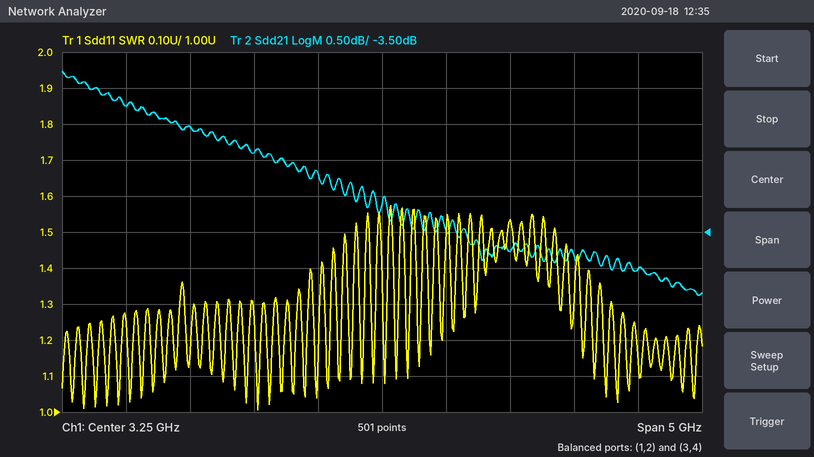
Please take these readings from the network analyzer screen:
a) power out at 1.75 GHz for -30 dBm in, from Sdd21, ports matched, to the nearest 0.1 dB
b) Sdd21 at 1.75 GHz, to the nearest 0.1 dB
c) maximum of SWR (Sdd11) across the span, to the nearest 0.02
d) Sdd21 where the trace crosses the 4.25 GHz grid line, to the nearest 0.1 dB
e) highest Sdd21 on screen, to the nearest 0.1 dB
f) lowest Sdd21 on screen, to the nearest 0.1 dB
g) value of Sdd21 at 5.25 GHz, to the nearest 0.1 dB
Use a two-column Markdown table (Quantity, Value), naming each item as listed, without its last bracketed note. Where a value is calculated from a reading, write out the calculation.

| Quantity | Value |
|---|---|
| power out at 1.75 GHz for -30 dBm in, from Sdd21, ports matched, to the nearest 0.1 dB | -30 dBm + (-2.0 dB) = -32.0 dBm |
| Sdd21 at 1.75 GHz, to the nearest 0.1 dB | -2.0 dB |
| maximum of SWR (Sdd11) across the span, to the nearest 0.02 | 1.58 |
| Sdd21 where the trace crosses the 4.25 GHz grid line, to the nearest 0.1 dB | -3.8 dB |
| highest Sdd21 on screen, to the nearest 0.1 dB | -1.3 dB |
| lowest Sdd21 on screen, to the nearest 0.1 dB | -4.4 dB |
| value of Sdd21 at 5.25 GHz, to the nearest 0.1 dB | -4.0 dB |
